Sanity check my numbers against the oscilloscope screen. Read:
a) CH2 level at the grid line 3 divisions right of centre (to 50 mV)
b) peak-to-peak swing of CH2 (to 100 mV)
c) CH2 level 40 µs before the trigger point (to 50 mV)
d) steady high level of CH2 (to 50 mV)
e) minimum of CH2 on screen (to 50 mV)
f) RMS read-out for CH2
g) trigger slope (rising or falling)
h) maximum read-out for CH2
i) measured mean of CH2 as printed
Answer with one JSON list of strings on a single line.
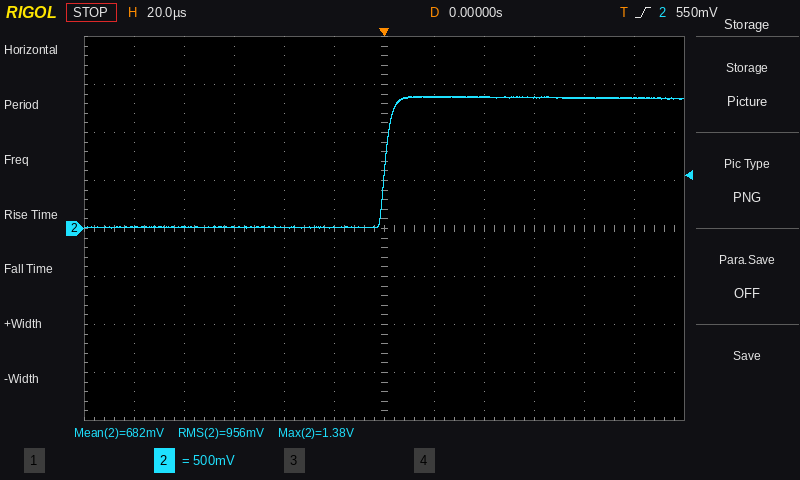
["1.35 V", "1.40 V", "0 mV", "1.35 V", "0 mV", "956 mV", "rising", "1.38 V", "682 mV"]
